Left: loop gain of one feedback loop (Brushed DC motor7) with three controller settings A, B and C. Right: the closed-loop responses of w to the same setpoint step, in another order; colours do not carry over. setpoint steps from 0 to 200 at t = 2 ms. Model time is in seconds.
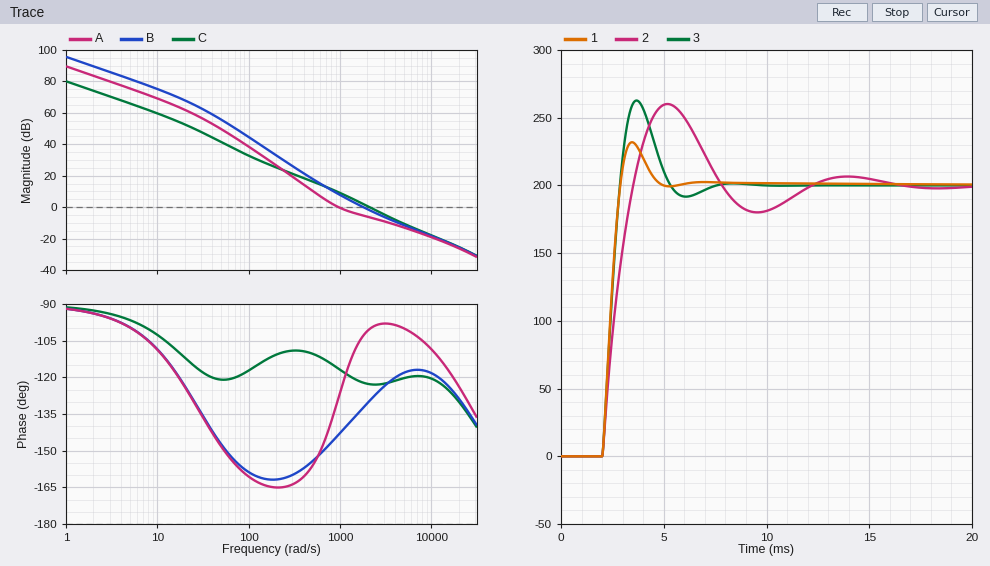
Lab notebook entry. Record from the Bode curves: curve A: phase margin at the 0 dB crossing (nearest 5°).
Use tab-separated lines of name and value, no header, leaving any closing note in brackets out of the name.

curve A: phase margin at the 0 dB crossing	50°
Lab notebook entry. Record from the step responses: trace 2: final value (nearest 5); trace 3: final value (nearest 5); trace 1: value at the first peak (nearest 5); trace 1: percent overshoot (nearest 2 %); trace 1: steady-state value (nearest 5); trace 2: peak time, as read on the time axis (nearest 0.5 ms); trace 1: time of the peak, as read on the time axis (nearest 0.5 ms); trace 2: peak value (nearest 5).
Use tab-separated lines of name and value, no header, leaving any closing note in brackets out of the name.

trace 2: final value	200
trace 3: final value	200
trace 1: value at the first peak	230
trace 1: percent overshoot	16 %
trace 1: steady-state value	200
trace 2: peak time, as read on the time axis	5.0 ms
trace 1: time of the peak, as read on the time axis	3.5 ms
trace 2: peak value	260
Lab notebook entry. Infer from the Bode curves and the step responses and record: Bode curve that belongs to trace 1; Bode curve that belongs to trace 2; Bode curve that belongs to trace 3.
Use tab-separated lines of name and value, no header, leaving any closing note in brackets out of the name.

Bode curve that belongs to trace 1	C
Bode curve that belongs to trace 2	A
Bode curve that belongs to trace 3	B
